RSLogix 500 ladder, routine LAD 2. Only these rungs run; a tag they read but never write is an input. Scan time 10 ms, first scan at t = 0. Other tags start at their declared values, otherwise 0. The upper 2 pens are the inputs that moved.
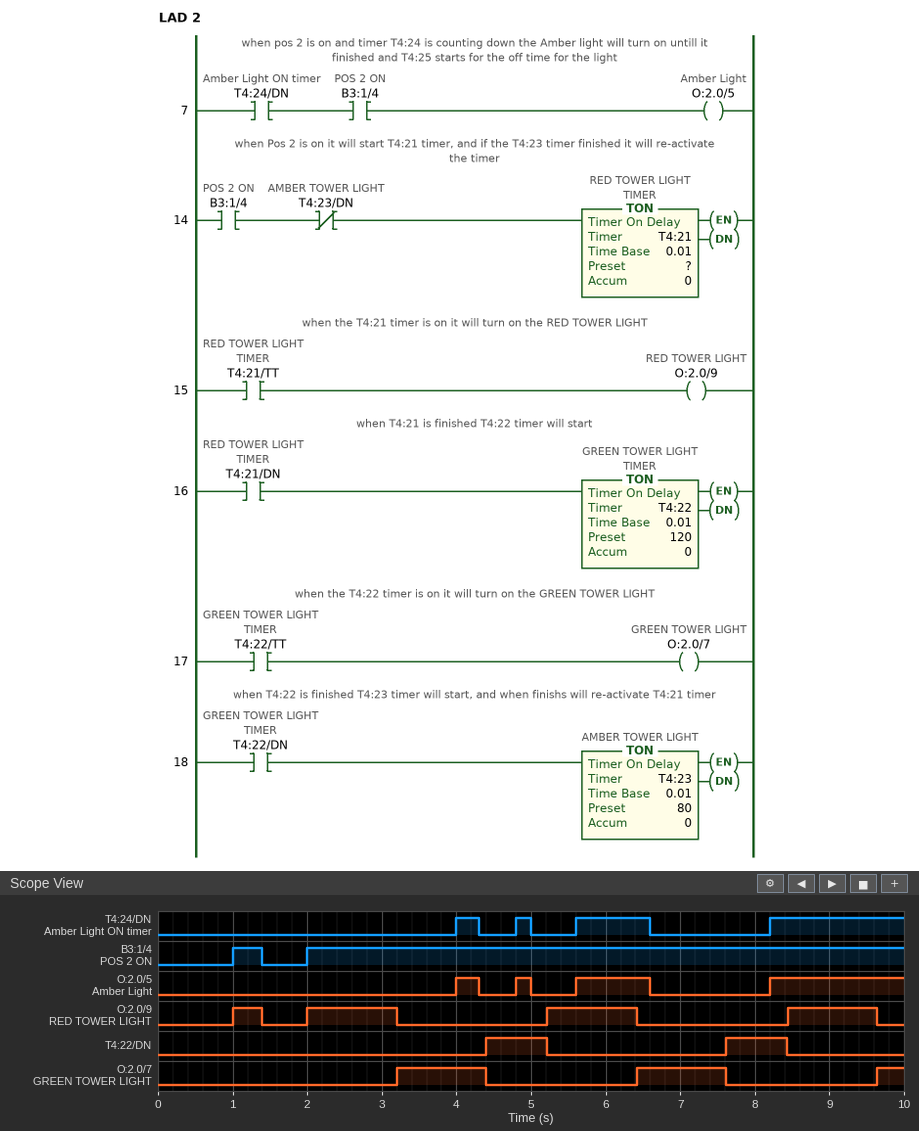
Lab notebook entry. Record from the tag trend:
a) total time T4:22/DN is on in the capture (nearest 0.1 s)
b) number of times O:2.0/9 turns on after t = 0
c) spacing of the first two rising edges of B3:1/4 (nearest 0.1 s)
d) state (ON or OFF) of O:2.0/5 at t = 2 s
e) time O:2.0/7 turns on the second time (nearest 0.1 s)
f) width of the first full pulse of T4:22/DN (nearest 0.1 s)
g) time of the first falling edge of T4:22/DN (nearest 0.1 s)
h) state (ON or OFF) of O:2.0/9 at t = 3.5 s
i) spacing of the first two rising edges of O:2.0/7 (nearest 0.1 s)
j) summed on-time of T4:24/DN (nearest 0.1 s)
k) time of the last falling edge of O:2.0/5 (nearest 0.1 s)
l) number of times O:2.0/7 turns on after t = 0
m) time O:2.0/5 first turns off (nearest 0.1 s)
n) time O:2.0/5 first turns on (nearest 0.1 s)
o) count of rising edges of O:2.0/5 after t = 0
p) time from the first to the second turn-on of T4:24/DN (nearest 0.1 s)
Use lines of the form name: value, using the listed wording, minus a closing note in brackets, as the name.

total time T4:22/DN is on in the capture: 1.6 s
number of times O:2.0/9 turns on after t = 0: 4
spacing of the first two rising edges of B3:1/4: 1.0 s
state (ON or OFF) of O:2.0/5 at t = 2 s: OFF
time O:2.0/7 turns on the second time: 6.4 s
width of the first full pulse of T4:22/DN: 0.8 s
time of the first falling edge of T4:22/DN: 5.2 s
state (ON or OFF) of O:2.0/9 at t = 3.5 s: OFF
spacing of the first two rising edges of O:2.0/7: 3.2 s
summed on-time of T4:24/DN: 3.3 s
time of the last falling edge of O:2.0/5: 6.6 s
number of times O:2.0/7 turns on after t = 0: 3
time O:2.0/5 first turns off: 4.3 s
time O:2.0/5 first turns on: 4.0 s
count of rising edges of O:2.0/5 after t = 0: 4
time from the first to the second turn-on of T4:24/DN: 0.8 s
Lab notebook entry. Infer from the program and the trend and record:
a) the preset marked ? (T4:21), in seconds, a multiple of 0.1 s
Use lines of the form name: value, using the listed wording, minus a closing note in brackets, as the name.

the preset marked ? (T4:21), in seconds, a multiple of 0.1 s: 1.2 s
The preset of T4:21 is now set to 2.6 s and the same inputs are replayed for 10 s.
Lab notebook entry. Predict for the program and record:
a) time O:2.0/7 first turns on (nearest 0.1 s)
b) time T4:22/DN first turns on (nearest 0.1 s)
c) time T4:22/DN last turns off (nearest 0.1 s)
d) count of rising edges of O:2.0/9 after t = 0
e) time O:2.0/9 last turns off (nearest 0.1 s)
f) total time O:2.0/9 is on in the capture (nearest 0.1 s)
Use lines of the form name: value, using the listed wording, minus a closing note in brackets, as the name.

time O:2.0/7 first turns on: 4.6 s
time T4:22/DN first turns on: 5.8 s
time T4:22/DN last turns off: 6.6 s
count of rising edges of O:2.0/9 after t = 0: 3
time O:2.0/9 last turns off: 9.2 s
total time O:2.0/9 is on in the capture: 5.6 s
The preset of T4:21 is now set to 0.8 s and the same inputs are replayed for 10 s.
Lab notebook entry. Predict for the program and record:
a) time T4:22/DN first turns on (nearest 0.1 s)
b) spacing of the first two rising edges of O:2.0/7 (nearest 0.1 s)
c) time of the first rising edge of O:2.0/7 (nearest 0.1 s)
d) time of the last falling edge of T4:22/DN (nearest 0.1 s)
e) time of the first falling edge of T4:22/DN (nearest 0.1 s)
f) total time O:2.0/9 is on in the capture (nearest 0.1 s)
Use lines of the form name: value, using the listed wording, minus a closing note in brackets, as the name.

time T4:22/DN first turns on: 4.0 s
spacing of the first two rising edges of O:2.0/7: 2.8 s
time of the first rising edge of O:2.0/7: 2.8 s
time of the last falling edge of T4:22/DN: 7.6 s
time of the first falling edge of T4:22/DN: 4.8 s
total time O:2.0/9 is on in the capture: 2.8 s
